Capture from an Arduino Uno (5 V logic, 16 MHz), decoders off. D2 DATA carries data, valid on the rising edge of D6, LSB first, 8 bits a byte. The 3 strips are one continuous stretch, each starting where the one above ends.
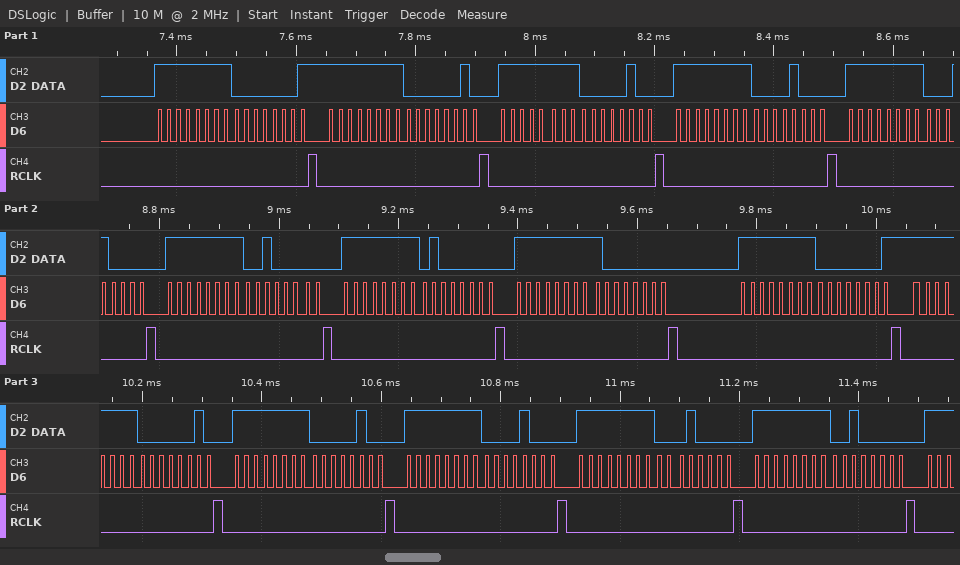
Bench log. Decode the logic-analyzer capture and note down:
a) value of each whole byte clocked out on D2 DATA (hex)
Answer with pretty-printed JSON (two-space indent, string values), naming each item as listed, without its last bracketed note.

{
  "value of each whole byte clocked out on D2 DATA": "FF 80 FF 40 FF 20 FF 10 FF 08 FF 04 FF 02 FF 01 FF 80 FF 40 FF 20 FF 10 FF 08 FF 04"
}
